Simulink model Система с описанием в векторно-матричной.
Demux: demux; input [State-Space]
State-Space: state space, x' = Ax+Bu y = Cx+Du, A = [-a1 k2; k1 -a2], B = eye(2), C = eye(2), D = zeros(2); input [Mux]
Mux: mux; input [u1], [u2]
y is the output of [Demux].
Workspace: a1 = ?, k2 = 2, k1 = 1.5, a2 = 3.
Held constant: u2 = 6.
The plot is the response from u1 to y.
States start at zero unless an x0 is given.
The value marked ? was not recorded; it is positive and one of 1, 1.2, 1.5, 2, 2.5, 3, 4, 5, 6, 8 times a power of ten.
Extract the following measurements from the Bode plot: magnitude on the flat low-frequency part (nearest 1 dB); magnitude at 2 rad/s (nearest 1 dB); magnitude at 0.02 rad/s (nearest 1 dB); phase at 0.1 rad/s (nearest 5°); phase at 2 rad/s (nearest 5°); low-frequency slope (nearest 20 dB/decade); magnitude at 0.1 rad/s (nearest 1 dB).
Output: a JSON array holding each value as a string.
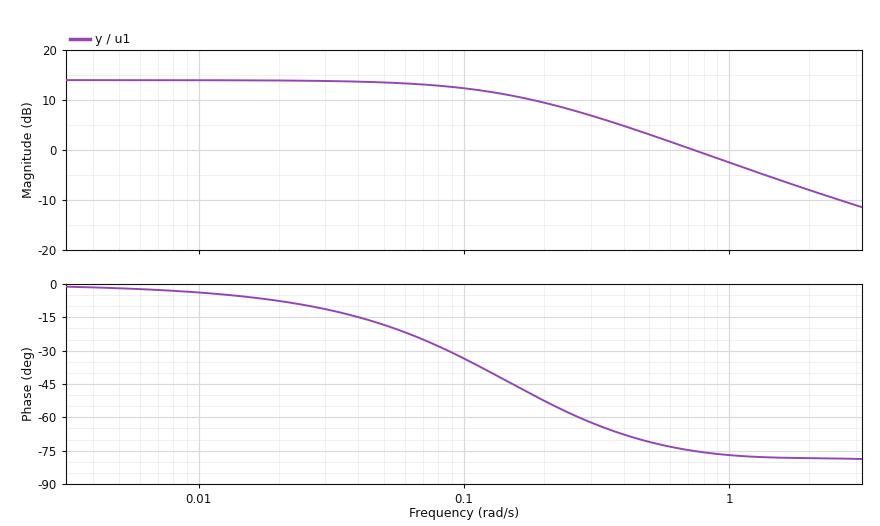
["14 dB", "-8 dB", "14 dB", "-35°", "-80°", "0 dB/decade", "12 dB"]
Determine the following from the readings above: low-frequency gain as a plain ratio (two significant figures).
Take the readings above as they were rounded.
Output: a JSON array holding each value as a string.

["5.0"]
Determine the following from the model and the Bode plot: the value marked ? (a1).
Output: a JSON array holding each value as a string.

["1.2"]
